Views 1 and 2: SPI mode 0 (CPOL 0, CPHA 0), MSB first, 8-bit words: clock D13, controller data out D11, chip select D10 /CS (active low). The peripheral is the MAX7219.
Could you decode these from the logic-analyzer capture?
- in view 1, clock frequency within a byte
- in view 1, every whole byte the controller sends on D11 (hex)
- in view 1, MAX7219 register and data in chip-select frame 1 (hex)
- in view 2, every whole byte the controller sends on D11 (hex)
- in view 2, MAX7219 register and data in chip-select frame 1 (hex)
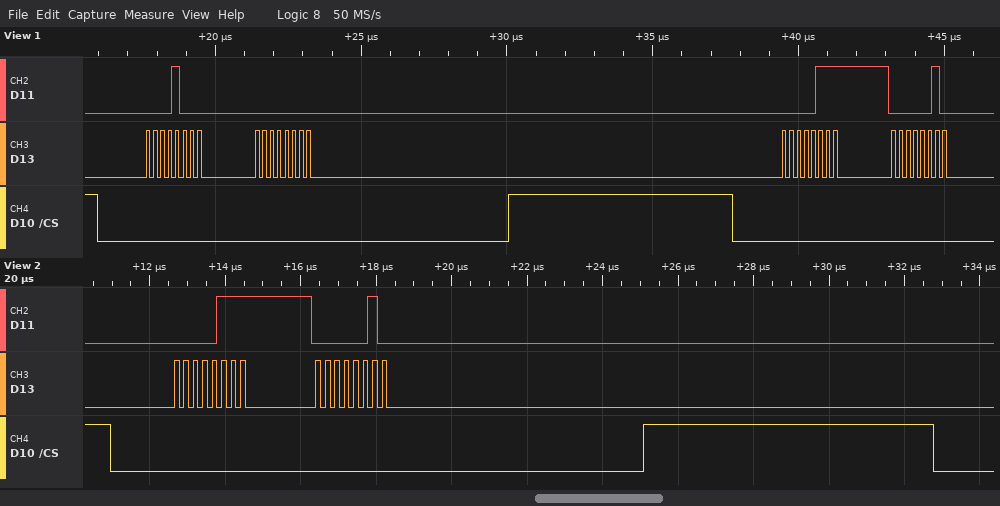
4 MHz
08 00 07 02
register 0x8, data 0x00
07 02
register 0x7, data 0x02
